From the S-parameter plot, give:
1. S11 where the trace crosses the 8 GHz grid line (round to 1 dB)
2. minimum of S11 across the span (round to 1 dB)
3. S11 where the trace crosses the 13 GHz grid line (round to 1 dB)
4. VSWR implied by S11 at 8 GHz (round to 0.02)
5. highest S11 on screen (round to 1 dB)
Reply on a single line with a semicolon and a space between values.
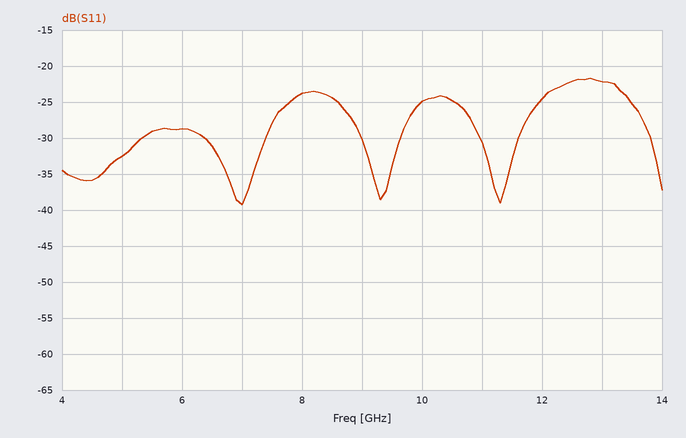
-24 dB; -39 dB; -22 dB; 1.14; -22 dB
